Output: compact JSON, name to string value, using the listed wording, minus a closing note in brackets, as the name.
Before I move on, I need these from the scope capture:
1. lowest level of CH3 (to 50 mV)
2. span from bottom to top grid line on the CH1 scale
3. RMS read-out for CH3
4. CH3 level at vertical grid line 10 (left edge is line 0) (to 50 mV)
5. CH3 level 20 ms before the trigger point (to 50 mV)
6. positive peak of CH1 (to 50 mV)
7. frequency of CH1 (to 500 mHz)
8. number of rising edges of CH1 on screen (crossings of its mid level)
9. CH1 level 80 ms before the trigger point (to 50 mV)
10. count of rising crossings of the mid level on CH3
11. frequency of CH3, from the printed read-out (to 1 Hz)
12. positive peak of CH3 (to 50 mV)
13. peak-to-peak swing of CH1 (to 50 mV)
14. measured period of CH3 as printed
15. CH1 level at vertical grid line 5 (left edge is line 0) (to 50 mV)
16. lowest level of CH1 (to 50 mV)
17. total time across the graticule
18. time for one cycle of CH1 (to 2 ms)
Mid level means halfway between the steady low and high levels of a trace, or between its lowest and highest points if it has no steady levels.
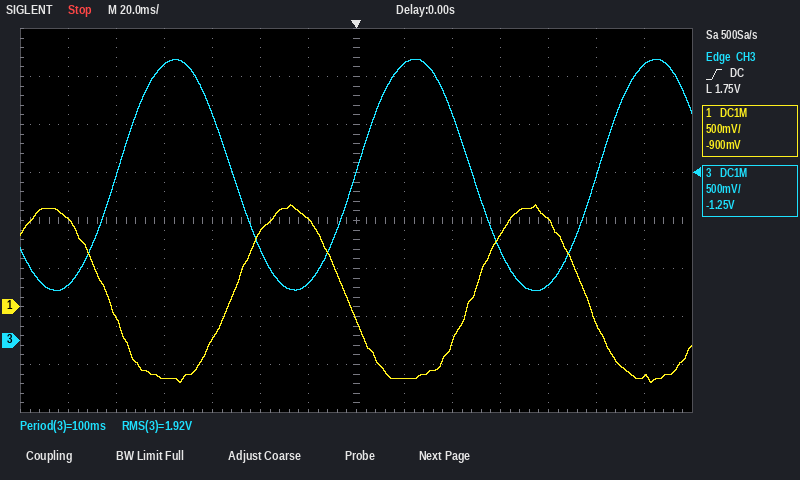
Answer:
{"lowest level of CH3": "500 mV", "span from bottom to top grid line on the CH1 scale": "4 V", "RMS read-out for CH3": "1.92 V", "CH3 level at vertical grid line 10 (left edge is line 0)": "950 mV", "CH3 level 20 ms before the trigger point": "600 mV", "positive peak of CH1": "1.05 V", "frequency of CH1": "10.0 Hz", "number of rising edges of CH1 on screen": "2", "CH1 level 80 ms before the trigger point": "-750 mV", "count of rising crossings of the mid level on CH3": "3", "frequency of CH3, from the printed read-out": "10 Hz", "positive peak of CH3": "2.95 V", "peak-to-peak swing of CH1": "1.85 V", "measured period of CH3 as printed": "100 ms", "CH1 level at vertical grid line 5 (left edge is line 0)": "800 mV", "lowest level of CH1": "-800 mV", "total time across the graticule": "280 ms", "time for one cycle of CH1": "100 ms"}
